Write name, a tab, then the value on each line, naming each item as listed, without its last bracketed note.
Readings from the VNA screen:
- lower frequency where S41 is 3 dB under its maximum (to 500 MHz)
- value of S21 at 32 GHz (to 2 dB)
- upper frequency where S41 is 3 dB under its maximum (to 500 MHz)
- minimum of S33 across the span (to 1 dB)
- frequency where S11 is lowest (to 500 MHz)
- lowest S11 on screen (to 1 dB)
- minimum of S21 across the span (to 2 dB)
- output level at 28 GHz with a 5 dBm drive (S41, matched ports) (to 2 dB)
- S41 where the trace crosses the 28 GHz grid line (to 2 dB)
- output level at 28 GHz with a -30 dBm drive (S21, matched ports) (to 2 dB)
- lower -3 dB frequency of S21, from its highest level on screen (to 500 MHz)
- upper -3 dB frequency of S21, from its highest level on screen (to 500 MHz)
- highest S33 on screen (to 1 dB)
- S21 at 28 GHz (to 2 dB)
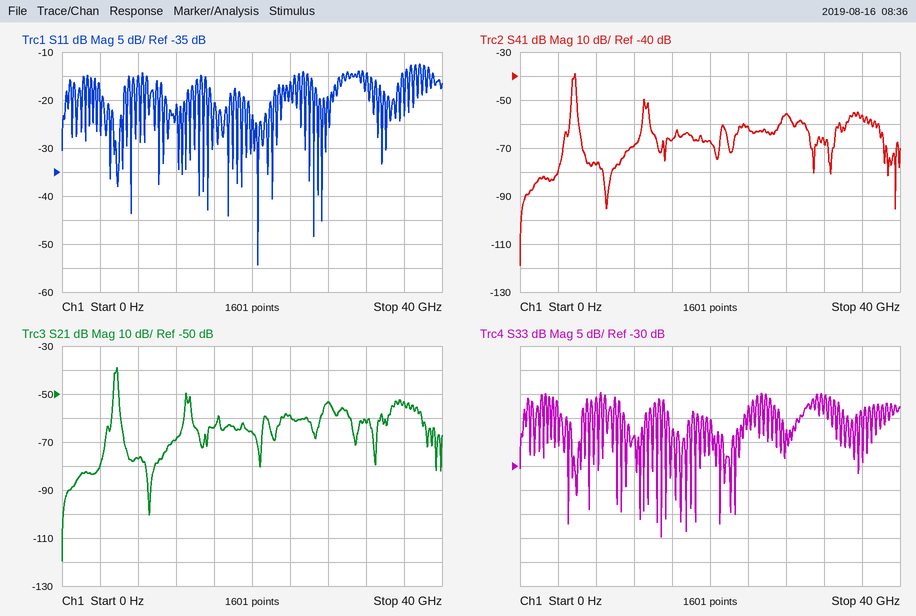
lower frequency where S41 is 3 dB under its maximum	5.5 GHz
value of S21 at 32 GHz	-62 dB
upper frequency where S41 is 3 dB under its maximum	6.0 GHz
minimum of S33 across the span	-45 dB
frequency where S11 is lowest	20.5 GHz
lowest S11 on screen	-54 dB
minimum of S21 across the span	-120 dB
output level at 28 GHz with a 5 dBm drive (S41, matched ports)	-50 dBm
S41 where the trace crosses the 28 GHz grid line	-56 dB
output level at 28 GHz with a -30 dBm drive (S21, matched ports)	-84 dBm
lower -3 dB frequency of S21, from its highest level on screen	5.5 GHz
upper -3 dB frequency of S21, from its highest level on screen	6.0 GHz
highest S33 on screen	-15 dB
S21 at 28 GHz	-54 dB
